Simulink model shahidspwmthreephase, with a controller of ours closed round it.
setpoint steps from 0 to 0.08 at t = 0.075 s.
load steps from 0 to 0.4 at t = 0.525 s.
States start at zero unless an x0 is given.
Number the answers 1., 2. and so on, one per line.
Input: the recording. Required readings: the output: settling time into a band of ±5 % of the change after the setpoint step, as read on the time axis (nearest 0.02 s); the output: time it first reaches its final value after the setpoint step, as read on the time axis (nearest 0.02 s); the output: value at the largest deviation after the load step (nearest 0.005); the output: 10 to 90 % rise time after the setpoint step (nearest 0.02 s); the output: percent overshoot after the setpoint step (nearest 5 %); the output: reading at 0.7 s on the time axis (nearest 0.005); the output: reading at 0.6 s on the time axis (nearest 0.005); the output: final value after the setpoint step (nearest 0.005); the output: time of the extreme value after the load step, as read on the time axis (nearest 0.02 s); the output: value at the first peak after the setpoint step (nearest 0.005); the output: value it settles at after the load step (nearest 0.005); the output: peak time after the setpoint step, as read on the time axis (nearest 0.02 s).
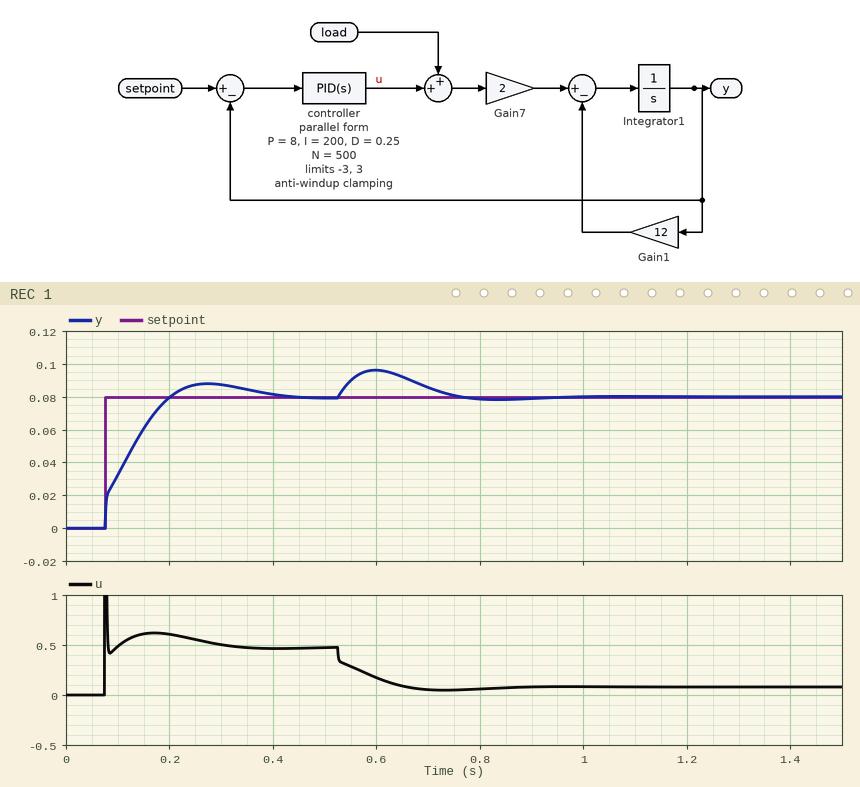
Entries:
1. 0.36 s
2. 0.20 s
3. 0.095
4. 0.10 s
5. 10 %
6. 0.085
7. 0.095
8. 0.080
9. 0.60 s
10. 0.090
11. 0.080
12. 0.28 s
